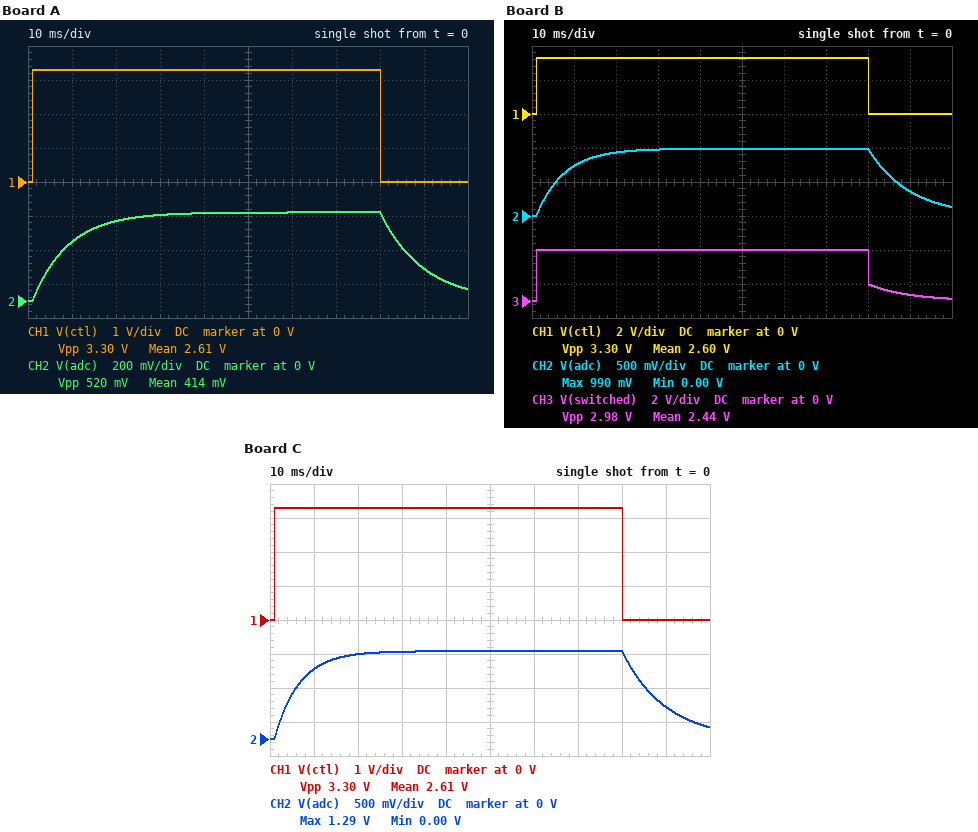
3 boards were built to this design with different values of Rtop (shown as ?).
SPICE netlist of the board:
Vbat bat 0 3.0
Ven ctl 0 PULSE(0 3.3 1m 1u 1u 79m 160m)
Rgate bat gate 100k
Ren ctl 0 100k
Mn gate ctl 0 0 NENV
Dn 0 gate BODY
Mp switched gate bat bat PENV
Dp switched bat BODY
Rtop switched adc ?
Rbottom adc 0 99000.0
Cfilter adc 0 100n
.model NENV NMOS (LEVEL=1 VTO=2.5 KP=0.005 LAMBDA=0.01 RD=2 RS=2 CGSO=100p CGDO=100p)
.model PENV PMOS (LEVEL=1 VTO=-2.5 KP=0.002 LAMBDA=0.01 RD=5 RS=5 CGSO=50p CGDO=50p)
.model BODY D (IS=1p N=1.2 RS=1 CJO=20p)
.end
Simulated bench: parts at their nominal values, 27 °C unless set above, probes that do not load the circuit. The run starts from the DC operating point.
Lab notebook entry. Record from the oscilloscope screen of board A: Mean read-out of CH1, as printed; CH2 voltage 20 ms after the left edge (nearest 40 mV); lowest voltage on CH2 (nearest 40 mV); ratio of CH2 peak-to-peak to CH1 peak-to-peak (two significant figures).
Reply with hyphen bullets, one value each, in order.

- 2.61 V
- 480 mV
- 0 V
- 0.16
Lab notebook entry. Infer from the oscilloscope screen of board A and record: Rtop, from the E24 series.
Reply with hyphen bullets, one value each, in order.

- 470 kΩ
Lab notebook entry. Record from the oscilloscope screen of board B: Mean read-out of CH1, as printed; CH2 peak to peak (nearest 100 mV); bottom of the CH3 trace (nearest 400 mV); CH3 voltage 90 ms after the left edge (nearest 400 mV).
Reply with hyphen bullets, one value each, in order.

- 2.60 V
- 1.0 V
- 0 V
- 400 mV
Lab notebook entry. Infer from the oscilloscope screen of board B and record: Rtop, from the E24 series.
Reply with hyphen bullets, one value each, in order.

- 200 kΩ
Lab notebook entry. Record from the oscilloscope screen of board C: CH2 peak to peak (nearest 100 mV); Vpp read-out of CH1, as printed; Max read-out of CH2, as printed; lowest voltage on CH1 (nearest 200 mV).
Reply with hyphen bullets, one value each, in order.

- 1.3 V
- 3.30 V
- 1.29 V
- 0 V
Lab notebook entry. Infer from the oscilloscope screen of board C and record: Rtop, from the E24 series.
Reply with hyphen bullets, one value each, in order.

- 130 kΩ
